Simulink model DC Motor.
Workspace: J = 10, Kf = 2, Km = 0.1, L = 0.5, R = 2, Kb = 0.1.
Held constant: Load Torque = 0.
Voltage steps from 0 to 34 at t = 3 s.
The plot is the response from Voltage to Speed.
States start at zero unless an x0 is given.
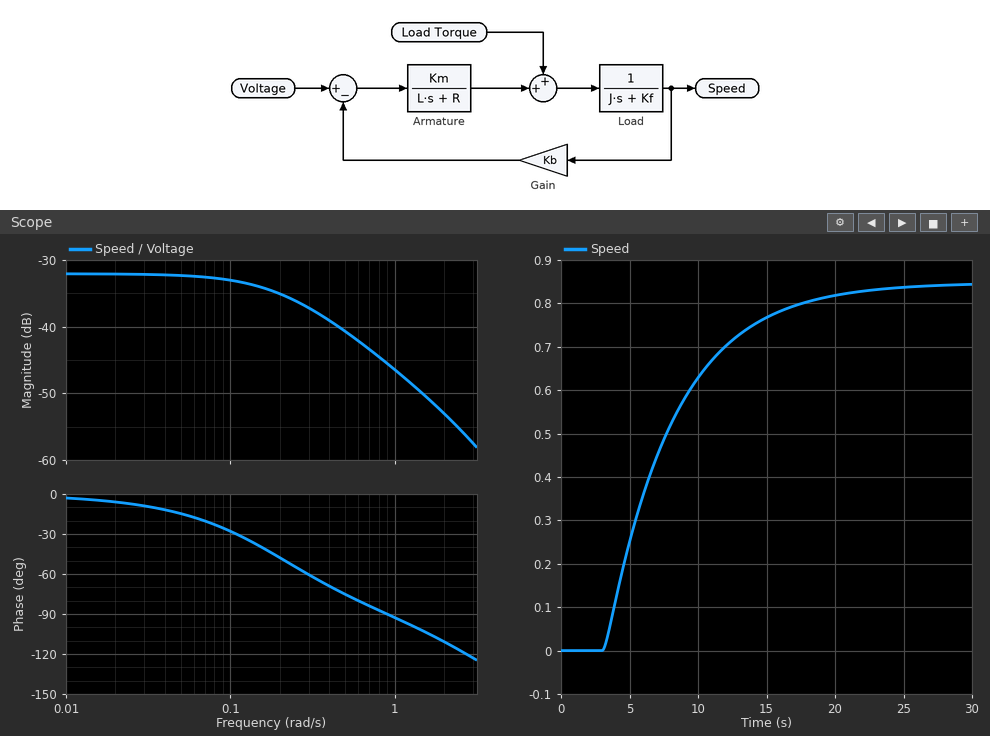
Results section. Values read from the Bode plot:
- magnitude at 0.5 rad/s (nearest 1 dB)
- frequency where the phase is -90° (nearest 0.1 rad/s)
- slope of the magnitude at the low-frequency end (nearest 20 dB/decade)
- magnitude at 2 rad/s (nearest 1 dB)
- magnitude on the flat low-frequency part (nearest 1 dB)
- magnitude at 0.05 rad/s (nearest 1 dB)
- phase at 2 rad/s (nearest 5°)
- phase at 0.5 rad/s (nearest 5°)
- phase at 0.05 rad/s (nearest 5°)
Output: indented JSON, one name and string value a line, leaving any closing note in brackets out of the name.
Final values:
{
  "magnitude at 0.5 rad/s": "-41 dB",
  "frequency where the phase is -90°": "0.9 rad/s",
  "slope of the magnitude at the low-frequency end": "0 dB/decade",
  "magnitude at 2 rad/s": "-53 dB",
  "magnitude on the flat low-frequency part": "-32 dB",
  "magnitude at 0.05 rad/s": "-32 dB",
  "phase at 2 rad/s": "-110°",
  "phase at 0.5 rad/s": "-75°",
  "phase at 0.05 rad/s": "-15°"
}
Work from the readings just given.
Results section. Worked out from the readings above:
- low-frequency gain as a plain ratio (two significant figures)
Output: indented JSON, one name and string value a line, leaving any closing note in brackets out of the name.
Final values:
{
  "low-frequency gain as a plain ratio": "0.025"
}
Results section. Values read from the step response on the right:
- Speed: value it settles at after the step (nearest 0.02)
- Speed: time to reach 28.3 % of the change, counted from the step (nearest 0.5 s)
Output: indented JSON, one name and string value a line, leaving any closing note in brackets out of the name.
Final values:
{
  "Speed: value it settles at after the step": "0.84",
  "Speed: time to reach 28.3 % of the change, counted from the step": "2.0 s"
}
